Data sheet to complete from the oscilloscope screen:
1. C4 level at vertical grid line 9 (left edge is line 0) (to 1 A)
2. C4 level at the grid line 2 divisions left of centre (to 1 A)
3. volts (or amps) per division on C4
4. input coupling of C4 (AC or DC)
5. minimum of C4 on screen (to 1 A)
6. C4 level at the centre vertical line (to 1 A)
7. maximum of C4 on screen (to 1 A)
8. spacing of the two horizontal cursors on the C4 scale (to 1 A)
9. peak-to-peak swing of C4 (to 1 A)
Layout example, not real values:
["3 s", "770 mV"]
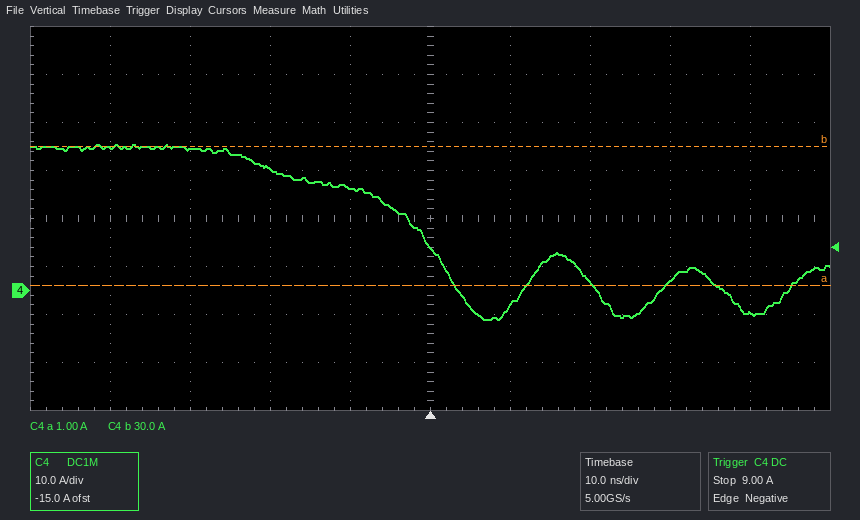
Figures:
["-5 A", "25 A", "10 A", "DC", "-6 A", "9 A", "30 A", "29 A", "36 A"]
